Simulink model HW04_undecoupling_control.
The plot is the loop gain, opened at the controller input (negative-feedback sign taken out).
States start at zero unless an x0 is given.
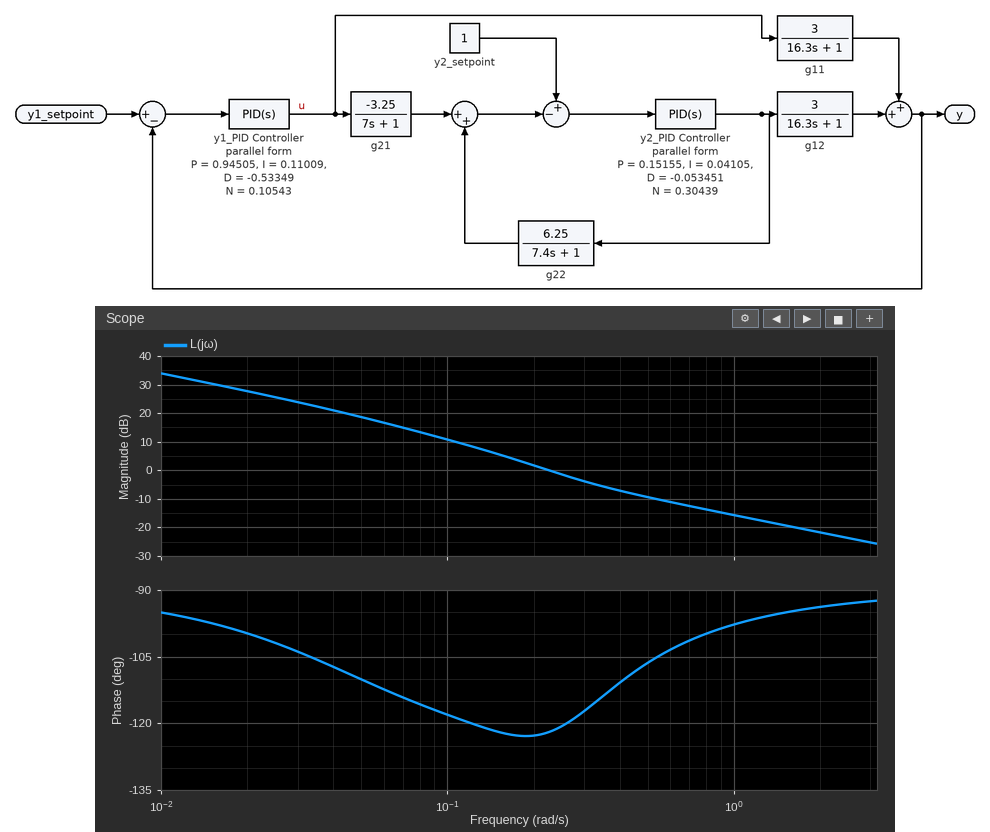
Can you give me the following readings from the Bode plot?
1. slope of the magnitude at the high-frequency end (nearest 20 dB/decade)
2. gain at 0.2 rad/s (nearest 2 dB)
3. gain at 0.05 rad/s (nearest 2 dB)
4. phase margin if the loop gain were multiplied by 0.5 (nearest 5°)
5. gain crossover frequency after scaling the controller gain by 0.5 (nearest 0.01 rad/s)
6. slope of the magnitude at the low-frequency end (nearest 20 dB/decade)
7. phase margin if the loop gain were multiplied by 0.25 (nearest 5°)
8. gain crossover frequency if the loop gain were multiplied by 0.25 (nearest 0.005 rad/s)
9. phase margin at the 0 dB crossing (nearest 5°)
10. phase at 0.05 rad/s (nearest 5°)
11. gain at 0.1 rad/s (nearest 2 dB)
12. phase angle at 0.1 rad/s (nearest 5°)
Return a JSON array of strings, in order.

["-20 dB/decade", "2 dB", "18 dB", "60°", "0.15 rad/s", "-20 dB/decade", "65°", "0.090 rad/s", "60°", "-110°", "10 dB", "-120°"]
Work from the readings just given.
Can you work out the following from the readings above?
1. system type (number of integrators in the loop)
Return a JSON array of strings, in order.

["1"]
